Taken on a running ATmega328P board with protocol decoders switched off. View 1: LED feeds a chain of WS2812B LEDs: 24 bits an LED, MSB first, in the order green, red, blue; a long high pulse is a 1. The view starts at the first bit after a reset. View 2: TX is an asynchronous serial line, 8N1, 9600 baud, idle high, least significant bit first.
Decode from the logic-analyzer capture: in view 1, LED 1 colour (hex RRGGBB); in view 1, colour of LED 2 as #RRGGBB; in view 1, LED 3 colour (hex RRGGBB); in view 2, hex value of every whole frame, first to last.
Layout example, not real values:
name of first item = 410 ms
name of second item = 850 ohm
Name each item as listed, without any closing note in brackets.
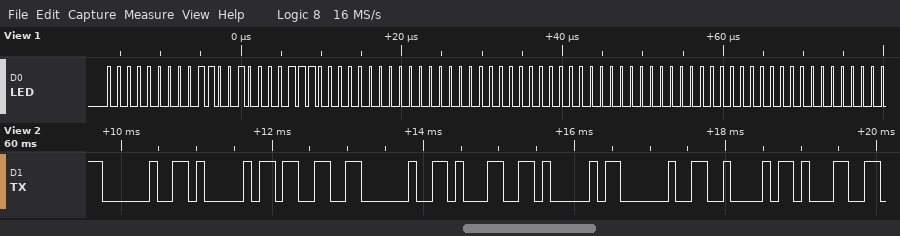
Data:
in view 1, LED 1 colour = #640038
in view 1, colour of LED 2 as #RRGGBB = #000000
in view 1, LED 3 colour = #000000
in view 2, hex value of every whole frame, first to last = 20 41 33 20 31 41 20 42 31
